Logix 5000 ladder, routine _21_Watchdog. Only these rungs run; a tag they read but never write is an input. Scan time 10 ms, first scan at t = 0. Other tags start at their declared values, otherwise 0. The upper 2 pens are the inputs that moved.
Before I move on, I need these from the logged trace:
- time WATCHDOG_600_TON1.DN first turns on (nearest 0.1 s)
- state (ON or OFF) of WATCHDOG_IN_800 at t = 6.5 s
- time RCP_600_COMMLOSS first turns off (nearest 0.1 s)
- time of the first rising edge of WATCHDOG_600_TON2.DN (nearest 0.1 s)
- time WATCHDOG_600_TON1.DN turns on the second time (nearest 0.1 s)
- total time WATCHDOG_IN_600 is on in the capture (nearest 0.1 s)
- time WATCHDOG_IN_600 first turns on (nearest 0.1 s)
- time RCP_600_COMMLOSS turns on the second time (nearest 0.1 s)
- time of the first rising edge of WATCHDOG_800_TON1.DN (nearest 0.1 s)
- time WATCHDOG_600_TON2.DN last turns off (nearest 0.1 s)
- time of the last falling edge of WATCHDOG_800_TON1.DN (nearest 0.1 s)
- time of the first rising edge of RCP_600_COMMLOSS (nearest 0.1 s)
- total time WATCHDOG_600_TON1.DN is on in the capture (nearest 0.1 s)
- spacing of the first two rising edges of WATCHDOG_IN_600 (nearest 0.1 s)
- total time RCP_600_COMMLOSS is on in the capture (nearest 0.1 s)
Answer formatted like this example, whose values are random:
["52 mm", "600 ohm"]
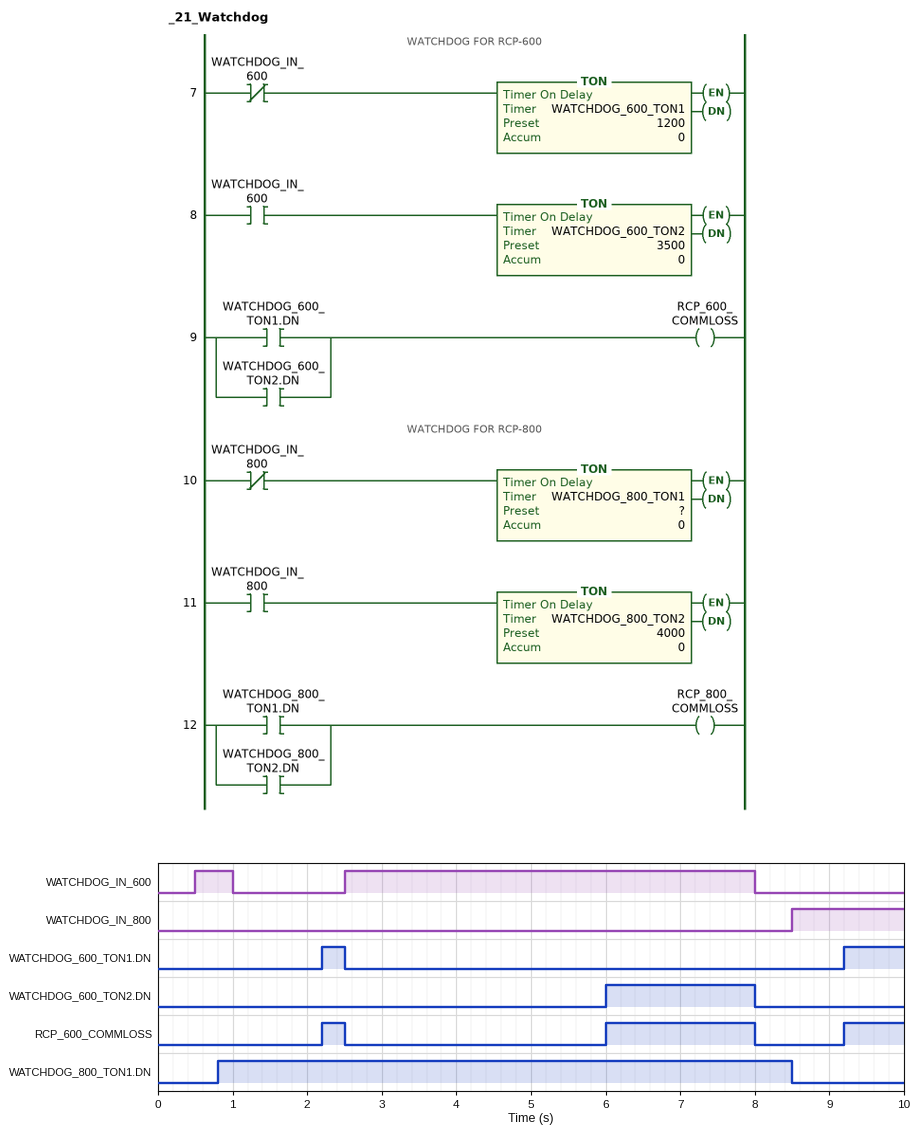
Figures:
["2.2 s", "OFF", "2.5 s", "6.0 s", "9.2 s", "6.0 s", "0.5 s", "6.0 s", "0.8 s", "8.0 s", "8.5 s", "2.2 s", "1.1 s", "2.0 s", "3.1 s"]
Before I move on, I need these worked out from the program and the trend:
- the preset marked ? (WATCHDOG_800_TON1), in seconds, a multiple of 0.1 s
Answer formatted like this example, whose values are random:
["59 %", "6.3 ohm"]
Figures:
["0.8 s"]
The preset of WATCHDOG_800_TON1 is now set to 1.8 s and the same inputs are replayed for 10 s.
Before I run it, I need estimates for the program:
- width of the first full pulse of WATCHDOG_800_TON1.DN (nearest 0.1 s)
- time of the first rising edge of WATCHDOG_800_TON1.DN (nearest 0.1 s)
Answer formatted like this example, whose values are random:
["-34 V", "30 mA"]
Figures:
["6.7 s", "1.8 s"]
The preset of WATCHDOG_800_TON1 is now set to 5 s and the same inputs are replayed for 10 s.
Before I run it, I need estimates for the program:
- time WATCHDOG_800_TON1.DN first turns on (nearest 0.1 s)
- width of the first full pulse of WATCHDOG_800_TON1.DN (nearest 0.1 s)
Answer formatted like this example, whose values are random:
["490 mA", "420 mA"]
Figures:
["5.0 s", "3.5 s"]
